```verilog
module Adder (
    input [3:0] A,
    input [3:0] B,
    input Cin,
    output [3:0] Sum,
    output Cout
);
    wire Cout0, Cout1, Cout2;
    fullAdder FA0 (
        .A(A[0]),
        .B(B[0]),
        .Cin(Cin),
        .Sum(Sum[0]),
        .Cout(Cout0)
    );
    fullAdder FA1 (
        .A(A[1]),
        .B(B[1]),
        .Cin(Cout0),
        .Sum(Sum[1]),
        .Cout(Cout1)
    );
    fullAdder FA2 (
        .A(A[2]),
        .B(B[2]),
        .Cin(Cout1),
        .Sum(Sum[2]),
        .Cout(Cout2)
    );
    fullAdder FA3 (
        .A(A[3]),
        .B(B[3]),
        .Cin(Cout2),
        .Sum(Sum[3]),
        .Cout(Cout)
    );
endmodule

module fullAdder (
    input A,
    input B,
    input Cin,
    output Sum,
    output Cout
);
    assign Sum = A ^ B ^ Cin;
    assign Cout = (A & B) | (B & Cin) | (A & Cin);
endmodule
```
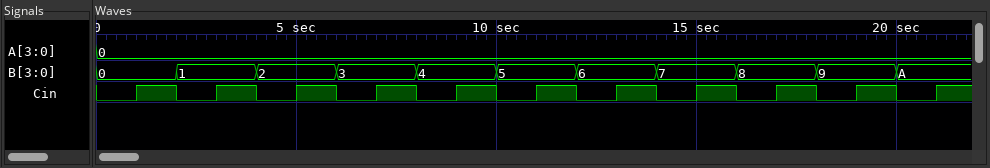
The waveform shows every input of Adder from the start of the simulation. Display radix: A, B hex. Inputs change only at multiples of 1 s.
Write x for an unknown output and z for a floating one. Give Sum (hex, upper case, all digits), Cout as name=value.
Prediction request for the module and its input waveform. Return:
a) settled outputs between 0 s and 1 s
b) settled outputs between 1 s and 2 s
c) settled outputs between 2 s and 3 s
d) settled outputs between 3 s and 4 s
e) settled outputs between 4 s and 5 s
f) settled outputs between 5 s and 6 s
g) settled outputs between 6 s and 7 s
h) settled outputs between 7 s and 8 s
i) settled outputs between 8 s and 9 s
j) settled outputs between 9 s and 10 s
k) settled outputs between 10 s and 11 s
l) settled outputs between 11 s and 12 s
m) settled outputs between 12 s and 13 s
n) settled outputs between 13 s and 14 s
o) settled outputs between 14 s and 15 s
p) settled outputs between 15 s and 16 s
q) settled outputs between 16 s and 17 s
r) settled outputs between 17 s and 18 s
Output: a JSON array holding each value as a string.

["Sum=0, Cout=0", "Sum=1, Cout=0", "Sum=1, Cout=0", "Sum=2, Cout=0", "Sum=2, Cout=0", "Sum=3, Cout=0", "Sum=3, Cout=0", "Sum=4, Cout=0", "Sum=4, Cout=0", "Sum=5, Cout=0", "Sum=5, Cout=0", "Sum=6, Cout=0", "Sum=6, Cout=0", "Sum=7, Cout=0", "Sum=7, Cout=0", "Sum=8, Cout=0", "Sum=8, Cout=0", "Sum=9, Cout=0"]
